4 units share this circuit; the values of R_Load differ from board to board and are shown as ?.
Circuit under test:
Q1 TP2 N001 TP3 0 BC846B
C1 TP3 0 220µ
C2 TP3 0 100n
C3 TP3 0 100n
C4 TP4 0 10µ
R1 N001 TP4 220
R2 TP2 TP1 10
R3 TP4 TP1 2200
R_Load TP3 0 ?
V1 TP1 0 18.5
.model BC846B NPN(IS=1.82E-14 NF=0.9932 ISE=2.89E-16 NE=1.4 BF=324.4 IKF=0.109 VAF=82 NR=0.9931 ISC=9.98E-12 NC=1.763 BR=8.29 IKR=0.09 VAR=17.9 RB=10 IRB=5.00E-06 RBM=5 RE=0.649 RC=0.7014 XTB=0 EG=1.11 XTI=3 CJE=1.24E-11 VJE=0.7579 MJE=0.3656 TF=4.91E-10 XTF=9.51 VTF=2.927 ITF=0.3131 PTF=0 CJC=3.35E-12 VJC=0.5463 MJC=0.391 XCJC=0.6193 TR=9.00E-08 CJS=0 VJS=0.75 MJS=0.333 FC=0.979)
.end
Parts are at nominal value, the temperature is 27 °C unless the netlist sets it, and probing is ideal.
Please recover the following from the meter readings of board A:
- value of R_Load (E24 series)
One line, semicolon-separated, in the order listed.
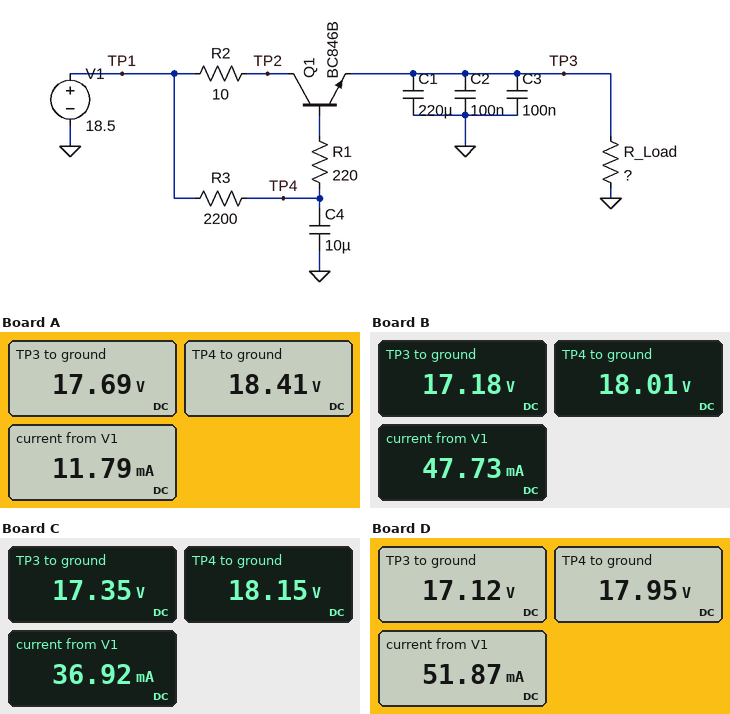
1.5 kΩ
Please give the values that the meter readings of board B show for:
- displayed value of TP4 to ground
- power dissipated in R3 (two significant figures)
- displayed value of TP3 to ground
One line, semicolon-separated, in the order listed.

18.01 V; 110 µW; 17.18 V
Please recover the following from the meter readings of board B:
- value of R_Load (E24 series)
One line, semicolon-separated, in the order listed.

360 Ω
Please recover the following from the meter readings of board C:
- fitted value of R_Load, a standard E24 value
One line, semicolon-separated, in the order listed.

470 Ω
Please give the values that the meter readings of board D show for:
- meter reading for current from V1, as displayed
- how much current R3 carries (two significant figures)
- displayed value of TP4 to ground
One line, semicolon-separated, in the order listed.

51.87 mA; 250 µA; 17.95 V
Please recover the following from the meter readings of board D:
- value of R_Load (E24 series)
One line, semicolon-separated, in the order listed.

330 Ω
